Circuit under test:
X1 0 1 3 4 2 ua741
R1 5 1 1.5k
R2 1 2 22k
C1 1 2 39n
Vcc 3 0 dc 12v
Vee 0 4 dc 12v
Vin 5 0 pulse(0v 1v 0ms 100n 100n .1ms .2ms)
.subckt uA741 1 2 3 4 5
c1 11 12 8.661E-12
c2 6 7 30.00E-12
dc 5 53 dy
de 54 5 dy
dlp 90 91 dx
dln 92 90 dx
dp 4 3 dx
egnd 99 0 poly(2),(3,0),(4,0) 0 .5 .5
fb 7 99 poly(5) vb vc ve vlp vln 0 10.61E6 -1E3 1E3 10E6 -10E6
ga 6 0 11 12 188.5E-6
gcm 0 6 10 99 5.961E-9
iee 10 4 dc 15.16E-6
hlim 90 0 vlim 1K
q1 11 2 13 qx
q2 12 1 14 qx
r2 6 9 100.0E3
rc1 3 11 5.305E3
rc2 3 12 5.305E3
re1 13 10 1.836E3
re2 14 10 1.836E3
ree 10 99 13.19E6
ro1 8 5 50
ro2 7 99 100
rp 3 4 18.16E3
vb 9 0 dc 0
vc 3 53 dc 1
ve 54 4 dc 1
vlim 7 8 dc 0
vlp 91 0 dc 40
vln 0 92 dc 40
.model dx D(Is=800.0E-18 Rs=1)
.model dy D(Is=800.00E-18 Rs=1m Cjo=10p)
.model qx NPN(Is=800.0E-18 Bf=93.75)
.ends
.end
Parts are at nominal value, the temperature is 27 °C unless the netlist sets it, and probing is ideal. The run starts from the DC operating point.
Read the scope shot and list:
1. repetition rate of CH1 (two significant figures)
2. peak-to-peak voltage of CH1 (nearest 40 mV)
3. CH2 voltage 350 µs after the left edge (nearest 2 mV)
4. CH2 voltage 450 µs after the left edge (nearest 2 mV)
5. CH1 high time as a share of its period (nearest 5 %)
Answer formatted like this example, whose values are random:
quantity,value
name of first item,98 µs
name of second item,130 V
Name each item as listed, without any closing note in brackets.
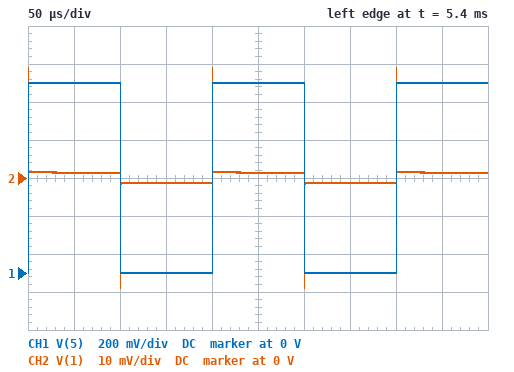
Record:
quantity,value
repetition rate of CH1,5.0 kHz
peak-to-peak voltage of CH1,1.00 V
CH2 voltage 350 µs after the left edge,-2 mV
CH2 voltage 450 µs after the left edge,2 mV
CH1 high time as a share of its period,50 %
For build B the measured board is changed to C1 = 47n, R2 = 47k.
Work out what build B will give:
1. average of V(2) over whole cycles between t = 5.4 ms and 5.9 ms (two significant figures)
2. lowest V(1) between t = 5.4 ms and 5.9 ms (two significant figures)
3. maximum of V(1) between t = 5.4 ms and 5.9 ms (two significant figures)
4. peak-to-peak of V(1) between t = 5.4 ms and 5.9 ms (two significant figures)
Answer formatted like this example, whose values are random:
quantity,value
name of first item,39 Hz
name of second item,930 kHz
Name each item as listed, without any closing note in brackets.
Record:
quantity,value
average of V(2) over whole cycles between t = 5.4 ms and 5.9 ms,-12 V
lowest V(1) between t = 5.4 ms and 5.9 ms,-20 mV
maximum of V(1) between t = 5.4 ms and 5.9 ms,390 mV
peak-to-peak of V(1) between t = 5.4 ms and 5.9 ms,410 mV
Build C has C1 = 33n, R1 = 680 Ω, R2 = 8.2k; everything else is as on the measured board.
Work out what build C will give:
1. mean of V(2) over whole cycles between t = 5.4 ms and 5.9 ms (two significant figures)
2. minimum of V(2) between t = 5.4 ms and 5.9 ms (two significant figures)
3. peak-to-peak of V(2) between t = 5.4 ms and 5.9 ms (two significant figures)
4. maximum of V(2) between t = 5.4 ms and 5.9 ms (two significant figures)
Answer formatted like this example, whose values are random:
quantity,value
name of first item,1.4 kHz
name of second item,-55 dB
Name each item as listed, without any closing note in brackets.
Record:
quantity,value
mean of V(2) over whole cycles between t = 5.4 ms and 5.9 ms,-6.0 V
minimum of V(2) between t = 5.4 ms and 5.9 ms,-7.2 V
peak-to-peak of V(2) between t = 5.4 ms and 5.9 ms,2.3 V
maximum of V(2) between t = 5.4 ms and 5.9 ms,-4.9 V
